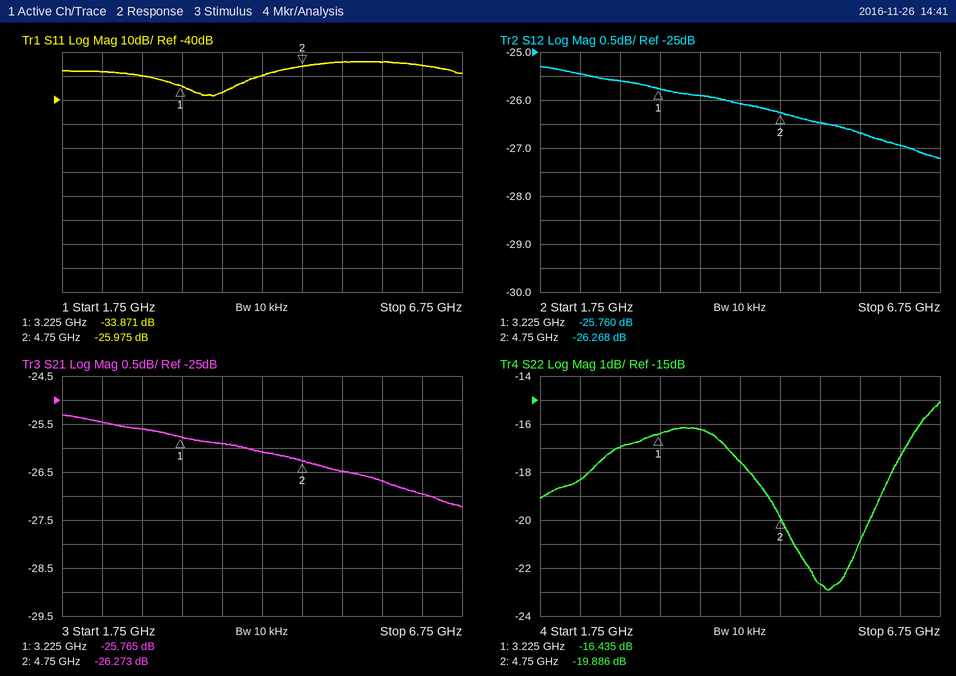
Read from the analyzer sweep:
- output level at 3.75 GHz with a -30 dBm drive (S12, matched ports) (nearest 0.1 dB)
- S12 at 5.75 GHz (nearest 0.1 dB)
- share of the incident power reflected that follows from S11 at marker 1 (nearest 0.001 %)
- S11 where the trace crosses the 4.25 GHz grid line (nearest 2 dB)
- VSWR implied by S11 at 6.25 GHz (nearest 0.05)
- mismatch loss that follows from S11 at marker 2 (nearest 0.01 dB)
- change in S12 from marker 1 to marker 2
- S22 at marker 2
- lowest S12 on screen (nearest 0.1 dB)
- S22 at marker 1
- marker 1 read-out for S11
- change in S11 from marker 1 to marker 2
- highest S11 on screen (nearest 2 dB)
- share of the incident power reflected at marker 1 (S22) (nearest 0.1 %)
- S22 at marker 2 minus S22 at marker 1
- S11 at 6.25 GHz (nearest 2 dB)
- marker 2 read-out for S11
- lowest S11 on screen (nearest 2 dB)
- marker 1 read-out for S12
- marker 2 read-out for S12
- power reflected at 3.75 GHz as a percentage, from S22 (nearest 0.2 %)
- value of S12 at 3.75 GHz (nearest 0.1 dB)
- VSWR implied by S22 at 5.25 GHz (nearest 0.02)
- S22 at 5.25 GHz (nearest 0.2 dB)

-55.9 dBm
-26.7 dB
0.041 %
-30 dB
1.10
0.01 dB
-0.508 dB
-19.886 dB
-27.2 dB
-16.435 dB
-33.871 dB
7.896 dB
-24 dB
2.3 %
-3.451 dB
-26 dB
-25.975 dB
-38 dB
-25.760 dB
-26.268 dB
2.4 %
-25.9 dB
1.16
-22.6 dB
